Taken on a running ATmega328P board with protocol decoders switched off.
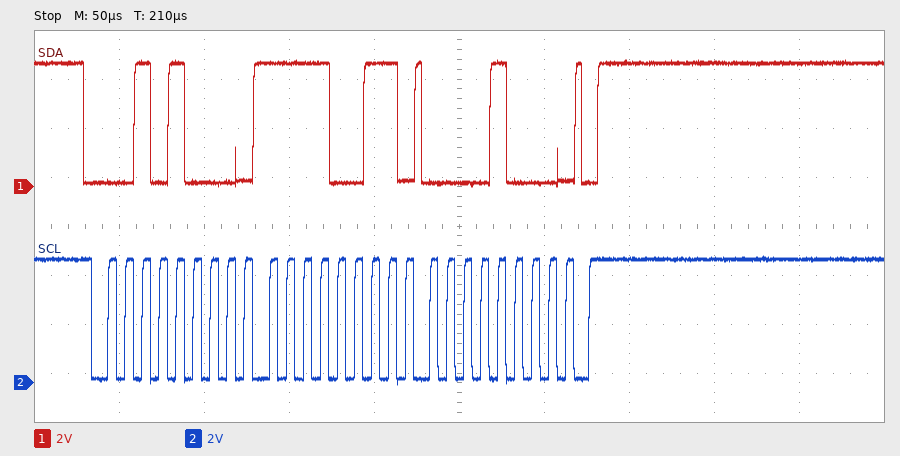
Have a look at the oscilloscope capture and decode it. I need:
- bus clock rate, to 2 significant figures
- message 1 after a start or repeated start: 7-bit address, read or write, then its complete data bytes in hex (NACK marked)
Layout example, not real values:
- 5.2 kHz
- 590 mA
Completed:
- 100 kHz
- 0x14 write: F3 08
